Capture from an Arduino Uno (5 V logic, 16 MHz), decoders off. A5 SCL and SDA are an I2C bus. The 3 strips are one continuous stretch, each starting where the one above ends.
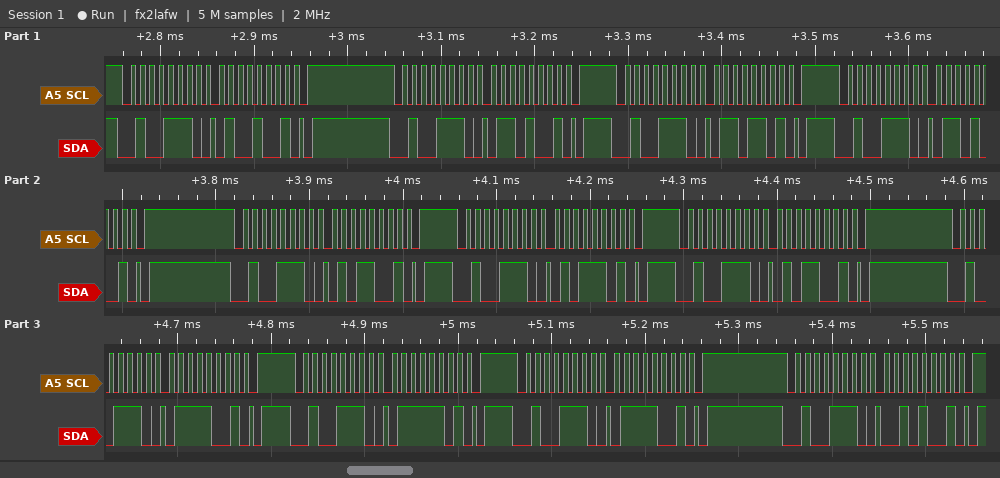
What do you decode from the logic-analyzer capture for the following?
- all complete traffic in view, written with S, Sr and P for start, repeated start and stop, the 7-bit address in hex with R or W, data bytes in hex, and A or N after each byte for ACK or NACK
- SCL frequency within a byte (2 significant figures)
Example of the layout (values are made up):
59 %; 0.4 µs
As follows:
S 27W A 49 A P S 27W A 69 A P S 27W A 6D A P S 27W A 69 A P S 27W A 59 A P S 27W A 5D A P S 27W A 59 A P S 27W A 79 A P S 27W A 7D A P S 27W A 79 A P S 27W A 29 A P; 100 kHz
